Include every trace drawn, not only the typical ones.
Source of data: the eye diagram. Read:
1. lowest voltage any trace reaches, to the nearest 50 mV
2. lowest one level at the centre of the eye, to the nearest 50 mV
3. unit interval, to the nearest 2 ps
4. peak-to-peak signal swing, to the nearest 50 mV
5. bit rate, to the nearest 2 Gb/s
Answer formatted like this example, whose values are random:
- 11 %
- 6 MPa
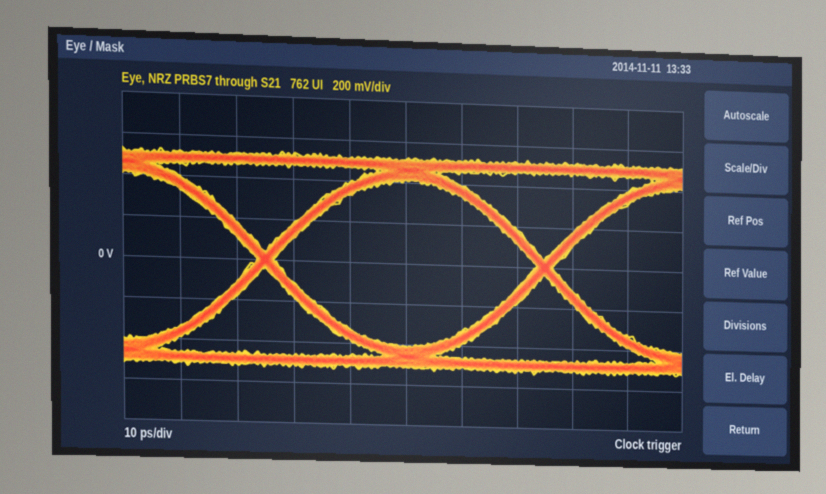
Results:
- -550 mV
- 400 mV
- 50 ps
- 1.05 V
- 20 Gb/s
